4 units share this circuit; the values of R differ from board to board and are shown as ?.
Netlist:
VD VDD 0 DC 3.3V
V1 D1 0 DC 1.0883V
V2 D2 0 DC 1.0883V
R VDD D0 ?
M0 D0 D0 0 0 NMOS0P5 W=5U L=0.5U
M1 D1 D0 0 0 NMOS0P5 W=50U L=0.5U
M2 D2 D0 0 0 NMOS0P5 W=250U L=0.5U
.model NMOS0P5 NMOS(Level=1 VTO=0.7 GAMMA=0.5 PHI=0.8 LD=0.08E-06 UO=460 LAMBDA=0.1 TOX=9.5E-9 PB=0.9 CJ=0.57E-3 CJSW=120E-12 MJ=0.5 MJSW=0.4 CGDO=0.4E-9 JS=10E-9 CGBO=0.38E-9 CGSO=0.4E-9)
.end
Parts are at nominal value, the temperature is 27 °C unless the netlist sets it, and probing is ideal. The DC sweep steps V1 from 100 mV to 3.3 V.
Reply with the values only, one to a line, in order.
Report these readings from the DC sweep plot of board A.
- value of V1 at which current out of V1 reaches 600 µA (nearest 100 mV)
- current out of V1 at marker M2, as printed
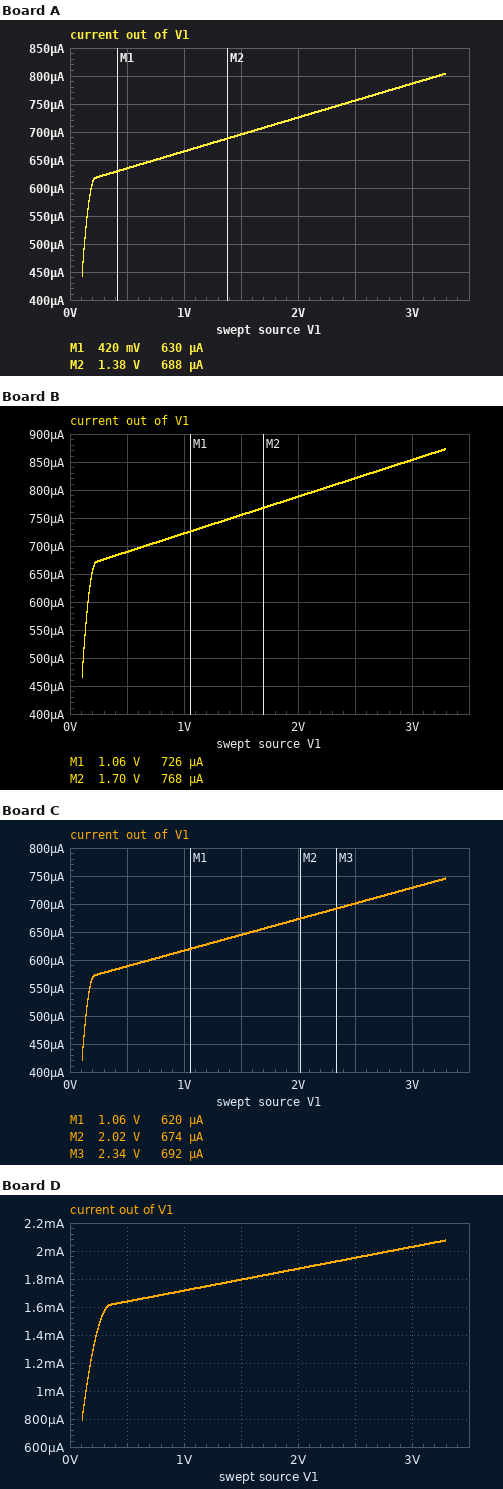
200 mV
688 µA
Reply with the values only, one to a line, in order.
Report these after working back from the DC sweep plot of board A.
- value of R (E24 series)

36 kΩ
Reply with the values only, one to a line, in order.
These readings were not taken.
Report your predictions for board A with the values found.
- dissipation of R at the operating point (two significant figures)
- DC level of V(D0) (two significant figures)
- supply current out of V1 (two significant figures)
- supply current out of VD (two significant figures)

160 µW
920 mV
670 µA
66 µA
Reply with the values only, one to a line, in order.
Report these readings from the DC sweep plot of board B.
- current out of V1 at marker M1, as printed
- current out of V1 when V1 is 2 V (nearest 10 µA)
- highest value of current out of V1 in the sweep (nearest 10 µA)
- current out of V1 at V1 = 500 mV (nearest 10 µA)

726 µA
790 µA
870 µA
690 µA
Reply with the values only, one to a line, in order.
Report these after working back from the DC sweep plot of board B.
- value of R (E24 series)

33 kΩ
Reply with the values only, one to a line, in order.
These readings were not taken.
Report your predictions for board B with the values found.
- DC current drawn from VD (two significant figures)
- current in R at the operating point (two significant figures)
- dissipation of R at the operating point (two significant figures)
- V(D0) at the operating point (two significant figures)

72 µA
72 µA
170 µW
930 mV
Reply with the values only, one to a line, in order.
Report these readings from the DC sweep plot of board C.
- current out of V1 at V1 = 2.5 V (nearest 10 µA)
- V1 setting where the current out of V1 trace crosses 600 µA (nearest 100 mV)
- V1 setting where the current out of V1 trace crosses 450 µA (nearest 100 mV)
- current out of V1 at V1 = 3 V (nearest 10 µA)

700 µA
700 mV
100 mV
730 µA
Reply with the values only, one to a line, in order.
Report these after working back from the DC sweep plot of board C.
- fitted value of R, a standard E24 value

39 kΩ
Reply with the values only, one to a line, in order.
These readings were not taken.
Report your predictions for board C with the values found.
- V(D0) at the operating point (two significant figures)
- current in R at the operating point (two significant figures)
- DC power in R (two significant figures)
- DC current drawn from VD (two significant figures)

910 mV
61 µA
150 µW
61 µA
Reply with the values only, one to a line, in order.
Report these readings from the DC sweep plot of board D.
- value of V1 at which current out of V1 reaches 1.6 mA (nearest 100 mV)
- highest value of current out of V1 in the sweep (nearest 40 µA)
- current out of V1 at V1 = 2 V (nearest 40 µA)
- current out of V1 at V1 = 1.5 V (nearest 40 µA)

300 mV
2.08 mA
1.88 mA
1.80 mA
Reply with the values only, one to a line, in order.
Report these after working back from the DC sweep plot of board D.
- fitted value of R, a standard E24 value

13 kΩ
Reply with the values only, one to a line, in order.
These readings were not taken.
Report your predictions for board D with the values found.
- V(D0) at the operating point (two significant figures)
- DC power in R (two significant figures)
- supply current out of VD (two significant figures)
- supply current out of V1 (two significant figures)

1.1 V
390 µW
170 µA
1.7 mA
